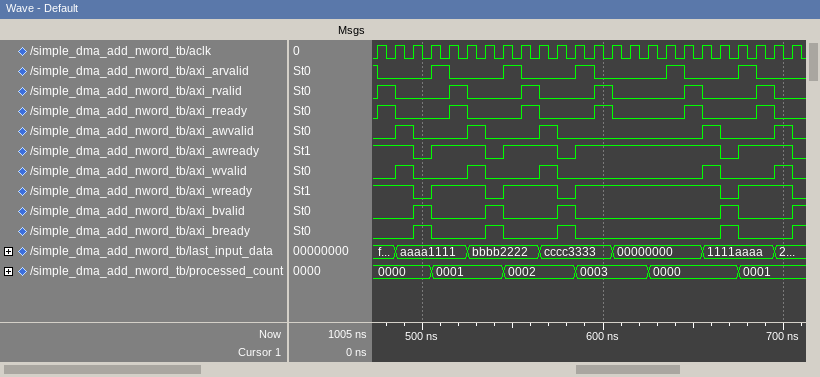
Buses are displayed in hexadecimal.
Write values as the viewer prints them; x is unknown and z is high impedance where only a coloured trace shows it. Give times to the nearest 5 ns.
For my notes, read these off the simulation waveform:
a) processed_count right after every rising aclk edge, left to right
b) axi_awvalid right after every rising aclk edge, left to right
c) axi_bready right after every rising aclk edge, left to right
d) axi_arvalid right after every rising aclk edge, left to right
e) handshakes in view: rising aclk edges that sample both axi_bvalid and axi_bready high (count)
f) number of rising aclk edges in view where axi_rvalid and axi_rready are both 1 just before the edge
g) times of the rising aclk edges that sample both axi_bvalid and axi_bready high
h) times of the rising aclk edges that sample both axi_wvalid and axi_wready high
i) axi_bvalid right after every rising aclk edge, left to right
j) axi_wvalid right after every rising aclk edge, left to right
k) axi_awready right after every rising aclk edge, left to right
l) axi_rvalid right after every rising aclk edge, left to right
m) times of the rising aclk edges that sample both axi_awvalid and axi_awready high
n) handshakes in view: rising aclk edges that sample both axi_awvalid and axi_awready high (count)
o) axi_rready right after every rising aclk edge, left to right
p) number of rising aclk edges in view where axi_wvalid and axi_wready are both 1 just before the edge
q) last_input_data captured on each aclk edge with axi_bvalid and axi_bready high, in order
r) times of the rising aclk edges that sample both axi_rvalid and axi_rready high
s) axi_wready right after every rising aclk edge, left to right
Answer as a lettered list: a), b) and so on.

a) 0000, 0000, 0000, 0001, 0001, 0001, 0001, 0002, 0002, 0002, 0002, 0003, 0003, 0003, 0003, 0000, 0000, 0000, 0000, 0000, 0001, 0001, 0001, 0001
b) 0 1 0 0 0 1 0 0 0 1 0 0 0 0 0 0 0 0 1 0 0 0 1 0
c) 0 0 1 0 0 0 1 0 0 0 1 0 0 0 0 0 0 0 0 1 0 0 0 1
d) 0 0 0 1 0 0 0 1 0 0 0 1 0 0 0 0 1 0 0 0 1 0 0 0
e) 4
f) 6
g) 505 ns, 545 ns, 585 ns, 675 ns
h) 495 ns, 535 ns, 575 ns, 665 ns, 705 ns
i) 0 0 1 0 0 0 1 0 0 0 1 0 0 0 0 0 0 0 0 1 0 0 0 1
j) 0 1 0 0 0 1 0 0 0 1 0 0 0 0 0 0 0 0 1 0 0 0 1 0
k) 1 1 0 1 1 1 0 1 1 1 0 1 1 1 1 1 1 1 1 0 1 1 1 0
l) 1 0 0 0 1 0 0 0 1 0 0 0 1 0 0 0 0 1 0 0 0 1 0 0
m) 495 ns, 535 ns, 575 ns, 665 ns, 705 ns
n) 5
o) 1 0 0 0 1 0 0 0 1 0 0 0 1 0 0 0 0 1 0 0 0 1 0 0
p) 5
q) aaaa1111, bbbb2222, cccc3333, 1111aaaa
r) 485 ns, 525 ns, 565 ns, 605 ns, 655 ns, 695 ns
s) 1 1 0 1 1 1 0 1 1 1 0 1 1 1 1 1 1 1 1 0 1 1 1 0
